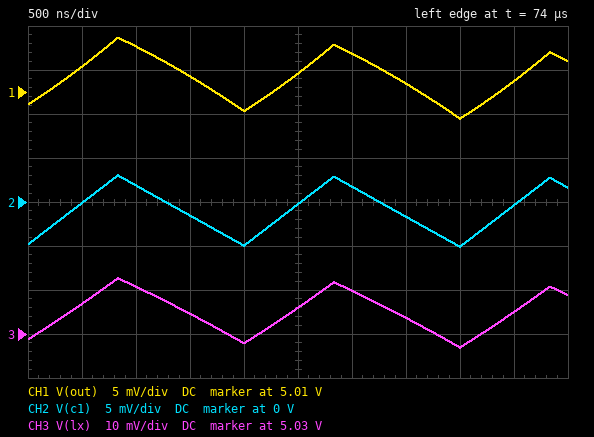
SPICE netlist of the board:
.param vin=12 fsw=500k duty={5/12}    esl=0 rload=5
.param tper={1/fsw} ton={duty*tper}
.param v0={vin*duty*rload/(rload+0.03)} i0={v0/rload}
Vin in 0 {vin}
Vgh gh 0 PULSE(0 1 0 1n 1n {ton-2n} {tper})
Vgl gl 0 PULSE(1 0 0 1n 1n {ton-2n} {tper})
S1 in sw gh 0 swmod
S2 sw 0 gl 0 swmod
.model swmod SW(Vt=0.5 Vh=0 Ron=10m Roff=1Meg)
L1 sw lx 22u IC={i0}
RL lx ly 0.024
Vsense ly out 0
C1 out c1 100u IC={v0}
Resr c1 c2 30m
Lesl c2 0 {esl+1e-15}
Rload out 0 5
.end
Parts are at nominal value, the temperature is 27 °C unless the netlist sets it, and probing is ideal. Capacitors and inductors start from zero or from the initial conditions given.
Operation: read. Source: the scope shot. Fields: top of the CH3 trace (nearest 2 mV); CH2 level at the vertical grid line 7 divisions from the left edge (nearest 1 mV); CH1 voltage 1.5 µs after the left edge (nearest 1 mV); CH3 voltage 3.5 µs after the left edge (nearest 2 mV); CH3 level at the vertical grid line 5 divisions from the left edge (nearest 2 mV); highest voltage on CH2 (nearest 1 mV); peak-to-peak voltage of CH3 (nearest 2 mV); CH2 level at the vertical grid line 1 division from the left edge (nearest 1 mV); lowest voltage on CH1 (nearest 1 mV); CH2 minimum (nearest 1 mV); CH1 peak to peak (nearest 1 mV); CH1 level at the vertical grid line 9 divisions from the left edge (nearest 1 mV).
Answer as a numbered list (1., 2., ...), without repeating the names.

1. 5.042 V
2. -2 mV
3. 5.012 V
4. 5.034 V
5. 5.036 V
6. 3 mV
7. 16 mV
8. 0 V
9. 5.007 V
10. -5 mV
11. 9 mV
12. 5.011 V
